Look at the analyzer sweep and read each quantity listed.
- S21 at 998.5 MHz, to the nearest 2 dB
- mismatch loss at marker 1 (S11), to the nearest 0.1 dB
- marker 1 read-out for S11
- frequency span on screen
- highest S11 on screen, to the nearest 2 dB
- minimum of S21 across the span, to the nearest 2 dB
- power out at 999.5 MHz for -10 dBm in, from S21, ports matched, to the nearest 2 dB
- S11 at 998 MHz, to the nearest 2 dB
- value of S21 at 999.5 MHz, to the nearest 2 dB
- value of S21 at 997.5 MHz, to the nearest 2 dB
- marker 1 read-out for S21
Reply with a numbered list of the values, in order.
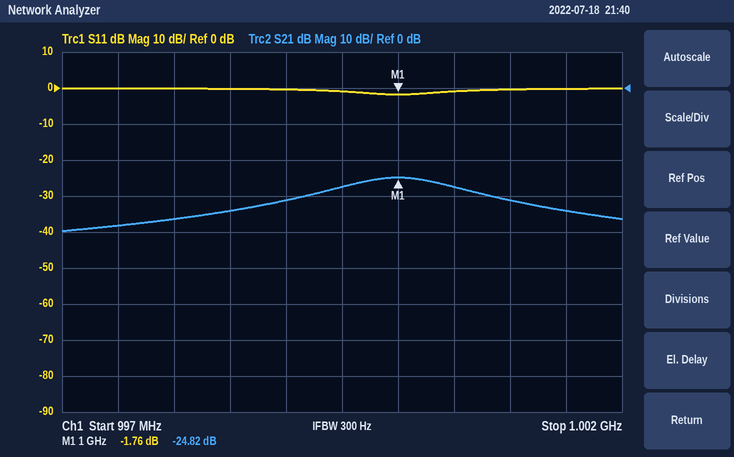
1. -34 dB
2. 4.8 dB
3. -1.76 dB
4. 5 MHz
5. 0 dB
6. -40 dB
7. -38 dBm
8. 0 dB
9. -28 dB
10. -38 dB
11. -24.82 dB
